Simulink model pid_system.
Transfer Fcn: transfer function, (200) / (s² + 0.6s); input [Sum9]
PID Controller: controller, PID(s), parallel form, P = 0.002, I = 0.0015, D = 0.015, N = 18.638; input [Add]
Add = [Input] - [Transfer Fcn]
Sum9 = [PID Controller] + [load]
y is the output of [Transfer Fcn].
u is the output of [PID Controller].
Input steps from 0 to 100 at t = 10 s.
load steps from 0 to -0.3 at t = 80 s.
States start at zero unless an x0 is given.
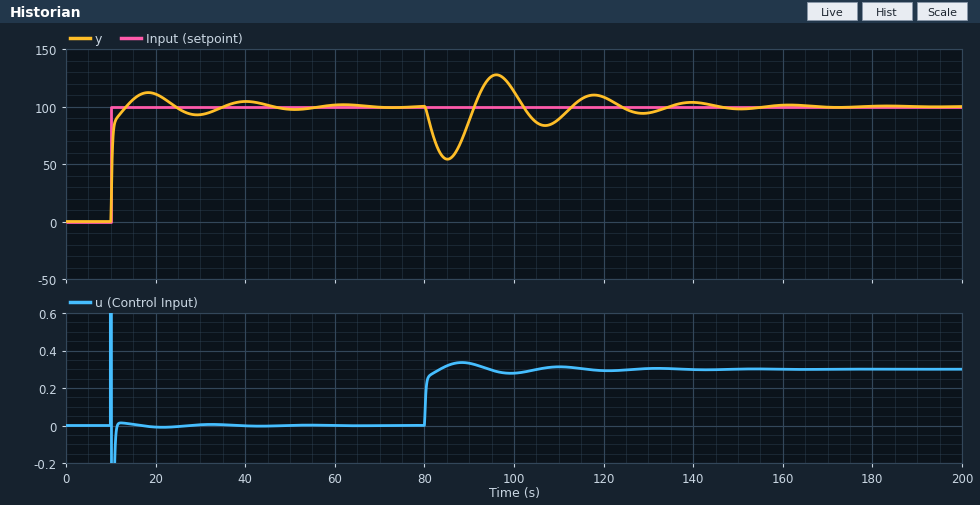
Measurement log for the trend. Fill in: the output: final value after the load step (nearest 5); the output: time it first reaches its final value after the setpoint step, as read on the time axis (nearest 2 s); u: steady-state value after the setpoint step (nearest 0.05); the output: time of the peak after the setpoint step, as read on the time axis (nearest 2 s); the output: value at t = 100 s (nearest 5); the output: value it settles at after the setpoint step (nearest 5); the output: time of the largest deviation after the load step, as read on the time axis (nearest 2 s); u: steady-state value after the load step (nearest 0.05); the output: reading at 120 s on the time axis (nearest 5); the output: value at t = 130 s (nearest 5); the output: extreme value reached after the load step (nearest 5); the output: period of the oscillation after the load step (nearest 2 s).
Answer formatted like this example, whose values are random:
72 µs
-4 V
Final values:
100
14 s
0.00
18 s
115
100
86 s
0.30
110
95
55
22 s
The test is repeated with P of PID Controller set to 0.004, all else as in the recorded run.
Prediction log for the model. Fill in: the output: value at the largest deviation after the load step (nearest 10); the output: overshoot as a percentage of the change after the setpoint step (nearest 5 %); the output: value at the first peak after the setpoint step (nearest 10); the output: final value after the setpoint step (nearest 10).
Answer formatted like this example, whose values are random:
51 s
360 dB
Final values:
60
10 %
110
100
